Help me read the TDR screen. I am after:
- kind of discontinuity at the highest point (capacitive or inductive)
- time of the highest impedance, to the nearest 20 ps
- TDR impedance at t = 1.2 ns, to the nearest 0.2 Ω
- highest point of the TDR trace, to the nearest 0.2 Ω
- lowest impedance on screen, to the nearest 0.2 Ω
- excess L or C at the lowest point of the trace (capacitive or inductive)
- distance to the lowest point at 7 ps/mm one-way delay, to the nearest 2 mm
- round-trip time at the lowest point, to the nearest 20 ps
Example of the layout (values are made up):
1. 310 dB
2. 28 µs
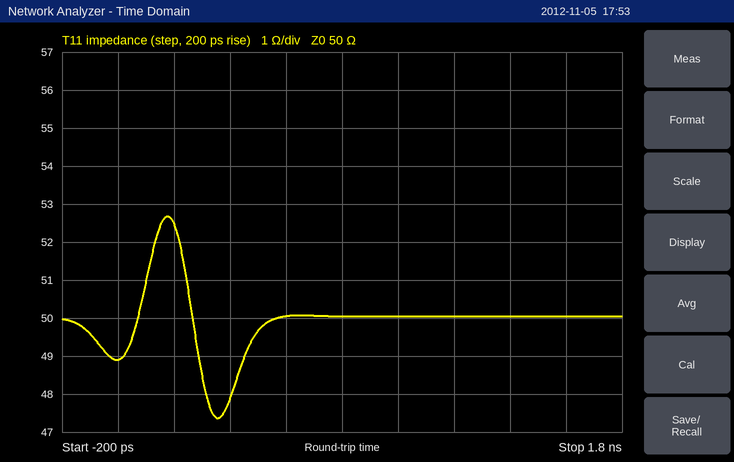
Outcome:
1. inductive
2. 180 ps
3. 50.0 Ω
4. 52.6 Ω
5. 47.4 Ω
6. capacitive
7. 26 mm
8. 360 ps
